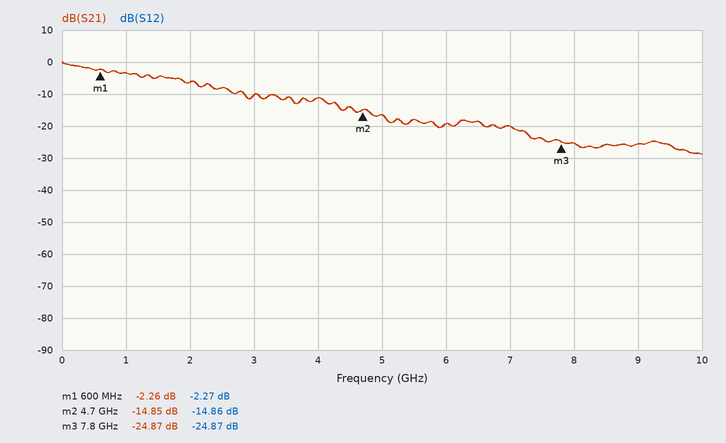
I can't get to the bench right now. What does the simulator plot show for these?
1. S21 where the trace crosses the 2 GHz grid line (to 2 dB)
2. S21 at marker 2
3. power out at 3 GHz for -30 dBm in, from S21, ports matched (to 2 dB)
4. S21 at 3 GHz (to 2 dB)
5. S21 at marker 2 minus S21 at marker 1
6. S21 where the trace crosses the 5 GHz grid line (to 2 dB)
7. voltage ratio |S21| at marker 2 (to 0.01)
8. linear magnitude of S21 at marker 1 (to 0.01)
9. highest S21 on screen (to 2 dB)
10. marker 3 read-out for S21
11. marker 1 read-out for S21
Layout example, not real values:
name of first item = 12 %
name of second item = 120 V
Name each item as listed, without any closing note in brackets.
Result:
S21 where the trace crosses the 2 GHz grid line = -6 dB
S21 at marker 2 = -14.85 dB
power out at 3 GHz for -30 dBm in, from S21, ports matched = -40 dBm
S21 at 3 GHz = -10 dB
S21 at marker 2 minus S21 at marker 1 = -12.59 dB
S21 where the trace crosses the 5 GHz grid line = -16 dB
voltage ratio |S21| at marker 2 = 0.18
linear magnitude of S21 at marker 1 = 0.77
highest S21 on screen = 0 dB
marker 3 read-out for S21 = -24.87 dB
marker 1 read-out for S21 = -2.26 dB
